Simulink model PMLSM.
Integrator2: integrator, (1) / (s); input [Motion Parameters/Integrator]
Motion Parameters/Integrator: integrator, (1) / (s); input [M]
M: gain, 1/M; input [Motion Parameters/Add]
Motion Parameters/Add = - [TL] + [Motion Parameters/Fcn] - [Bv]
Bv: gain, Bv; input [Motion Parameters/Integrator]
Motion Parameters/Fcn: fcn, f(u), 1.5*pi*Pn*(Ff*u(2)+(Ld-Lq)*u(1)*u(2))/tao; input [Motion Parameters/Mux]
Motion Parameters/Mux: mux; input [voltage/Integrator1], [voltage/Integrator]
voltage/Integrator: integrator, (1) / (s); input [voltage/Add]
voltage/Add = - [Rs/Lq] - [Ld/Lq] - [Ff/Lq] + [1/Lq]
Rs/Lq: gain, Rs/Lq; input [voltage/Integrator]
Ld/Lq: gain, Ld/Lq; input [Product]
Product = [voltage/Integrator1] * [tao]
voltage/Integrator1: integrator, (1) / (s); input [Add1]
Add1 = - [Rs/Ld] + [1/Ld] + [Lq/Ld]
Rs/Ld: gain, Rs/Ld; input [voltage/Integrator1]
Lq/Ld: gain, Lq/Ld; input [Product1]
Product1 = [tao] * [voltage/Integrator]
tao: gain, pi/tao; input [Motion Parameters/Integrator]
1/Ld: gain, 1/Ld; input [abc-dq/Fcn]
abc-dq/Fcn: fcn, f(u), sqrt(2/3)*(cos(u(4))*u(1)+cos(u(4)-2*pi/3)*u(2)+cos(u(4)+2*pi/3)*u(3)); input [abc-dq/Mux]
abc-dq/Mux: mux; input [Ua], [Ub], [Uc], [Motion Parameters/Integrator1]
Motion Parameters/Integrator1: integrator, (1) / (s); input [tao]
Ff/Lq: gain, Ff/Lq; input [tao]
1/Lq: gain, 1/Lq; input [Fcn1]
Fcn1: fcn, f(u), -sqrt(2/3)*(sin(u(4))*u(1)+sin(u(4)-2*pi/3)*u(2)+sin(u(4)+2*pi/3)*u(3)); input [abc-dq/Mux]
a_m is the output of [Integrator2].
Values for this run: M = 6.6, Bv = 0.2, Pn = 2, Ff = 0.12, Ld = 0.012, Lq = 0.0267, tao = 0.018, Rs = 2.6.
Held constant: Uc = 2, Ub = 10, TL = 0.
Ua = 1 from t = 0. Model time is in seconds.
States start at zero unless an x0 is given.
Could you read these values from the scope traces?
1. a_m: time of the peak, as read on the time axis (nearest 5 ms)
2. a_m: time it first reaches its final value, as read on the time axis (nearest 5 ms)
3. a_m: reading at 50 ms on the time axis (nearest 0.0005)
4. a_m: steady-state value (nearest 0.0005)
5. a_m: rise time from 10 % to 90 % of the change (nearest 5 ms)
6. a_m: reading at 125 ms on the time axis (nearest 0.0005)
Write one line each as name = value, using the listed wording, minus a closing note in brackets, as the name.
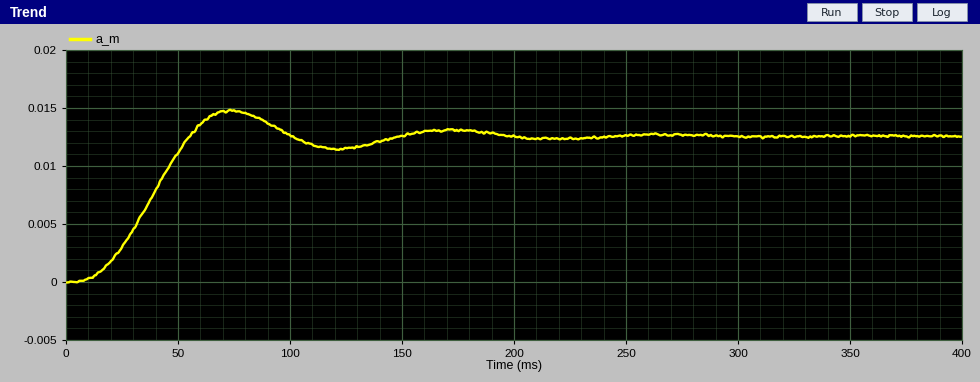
a_m: time of the peak, as read on the time axis = 75 ms
a_m: time it first reaches its final value, as read on the time axis = 55 ms
a_m: reading at 50 ms on the time axis = 0.0110
a_m: steady-state value = 0.0125
a_m: rise time from 10 % to 90 % of the change = 35 ms
a_m: reading at 125 ms on the time axis = 0.0115
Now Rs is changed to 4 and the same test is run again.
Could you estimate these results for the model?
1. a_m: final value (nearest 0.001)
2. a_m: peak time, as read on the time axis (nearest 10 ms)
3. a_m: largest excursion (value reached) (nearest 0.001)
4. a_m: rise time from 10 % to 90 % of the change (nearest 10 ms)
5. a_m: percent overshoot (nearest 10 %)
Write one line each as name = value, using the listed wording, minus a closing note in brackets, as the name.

a_m: final value = 0.013
a_m: peak time, as read on the time axis = 90 ms
a_m: largest excursion (value reached) = 0.015
a_m: rise time from 10 % to 90 % of the change = 40 ms
a_m: percent overshoot = 20 %
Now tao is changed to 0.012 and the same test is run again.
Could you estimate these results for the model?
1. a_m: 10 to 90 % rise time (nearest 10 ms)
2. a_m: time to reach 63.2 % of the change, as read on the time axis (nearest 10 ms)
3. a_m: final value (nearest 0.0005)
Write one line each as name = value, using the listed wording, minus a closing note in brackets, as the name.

a_m: 10 to 90 % rise time = 30 ms
a_m: time to reach 63.2 % of the change, as read on the time axis = 30 ms
a_m: final value = 0.0085
